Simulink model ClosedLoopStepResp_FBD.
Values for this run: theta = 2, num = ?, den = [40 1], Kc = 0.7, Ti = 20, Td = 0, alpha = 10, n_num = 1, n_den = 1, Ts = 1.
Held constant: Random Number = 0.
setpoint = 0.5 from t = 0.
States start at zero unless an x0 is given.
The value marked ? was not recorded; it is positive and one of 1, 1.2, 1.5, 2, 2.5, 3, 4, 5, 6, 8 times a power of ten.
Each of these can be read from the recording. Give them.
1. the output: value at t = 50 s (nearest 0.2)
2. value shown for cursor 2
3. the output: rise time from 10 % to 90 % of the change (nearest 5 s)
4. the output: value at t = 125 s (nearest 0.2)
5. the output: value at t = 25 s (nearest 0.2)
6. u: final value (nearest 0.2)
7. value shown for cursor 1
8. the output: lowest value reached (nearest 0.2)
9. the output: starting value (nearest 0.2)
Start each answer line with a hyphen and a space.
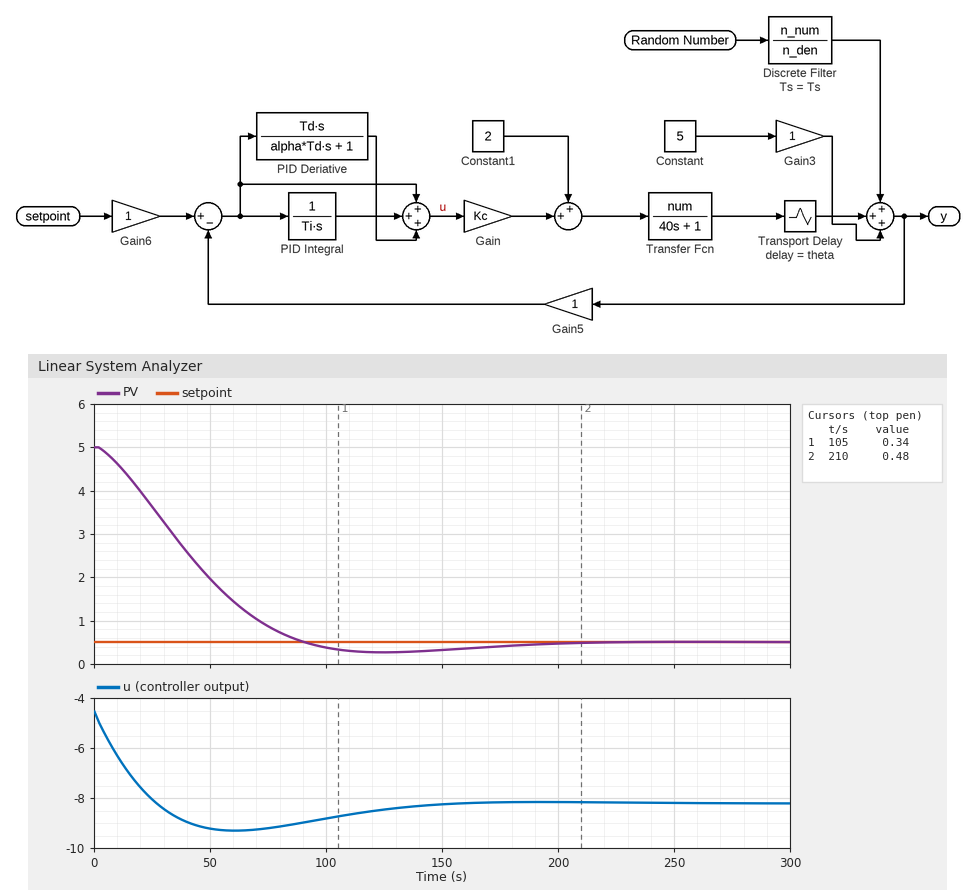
- 2.0
- 0.48
- 60 s
- 0.2
- 3.6
- -8.2
- 0.34
- 0.2
- 5.0
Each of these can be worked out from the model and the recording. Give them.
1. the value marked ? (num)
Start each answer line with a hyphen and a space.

- 1.2
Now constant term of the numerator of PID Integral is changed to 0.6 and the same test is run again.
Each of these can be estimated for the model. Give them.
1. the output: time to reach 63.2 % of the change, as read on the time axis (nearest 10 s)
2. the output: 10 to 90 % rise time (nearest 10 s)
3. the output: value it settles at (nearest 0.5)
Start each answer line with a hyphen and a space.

- 70 s
- 110 s
- 0.5
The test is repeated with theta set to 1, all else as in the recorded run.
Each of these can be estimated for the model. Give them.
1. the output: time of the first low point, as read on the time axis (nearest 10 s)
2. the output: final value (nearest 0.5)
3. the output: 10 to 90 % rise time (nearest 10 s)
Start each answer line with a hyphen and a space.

- 130 s
- 0.5
- 60 s
